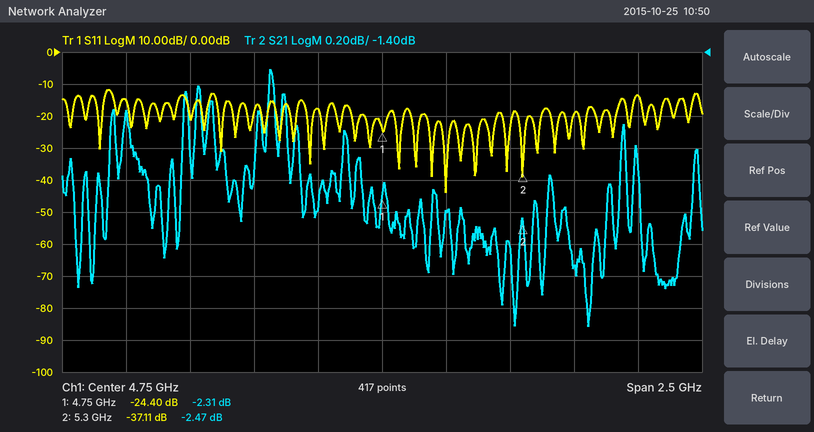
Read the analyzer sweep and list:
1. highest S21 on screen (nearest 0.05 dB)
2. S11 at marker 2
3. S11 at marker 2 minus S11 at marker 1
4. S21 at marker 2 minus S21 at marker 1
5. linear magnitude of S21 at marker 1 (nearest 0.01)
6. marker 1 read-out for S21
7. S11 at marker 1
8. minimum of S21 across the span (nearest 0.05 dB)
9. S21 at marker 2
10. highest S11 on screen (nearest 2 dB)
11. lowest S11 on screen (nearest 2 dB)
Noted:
-1.50 dB
-37.11 dB
-12.71 dB
-0.16 dB
0.77
-2.31 dB
-24.40 dB
-3.10 dB
-2.47 dB
-12 dB
-44 dB
